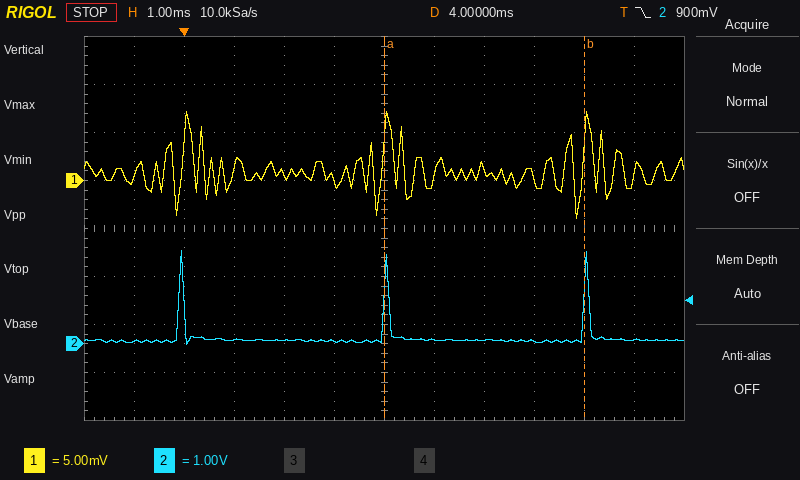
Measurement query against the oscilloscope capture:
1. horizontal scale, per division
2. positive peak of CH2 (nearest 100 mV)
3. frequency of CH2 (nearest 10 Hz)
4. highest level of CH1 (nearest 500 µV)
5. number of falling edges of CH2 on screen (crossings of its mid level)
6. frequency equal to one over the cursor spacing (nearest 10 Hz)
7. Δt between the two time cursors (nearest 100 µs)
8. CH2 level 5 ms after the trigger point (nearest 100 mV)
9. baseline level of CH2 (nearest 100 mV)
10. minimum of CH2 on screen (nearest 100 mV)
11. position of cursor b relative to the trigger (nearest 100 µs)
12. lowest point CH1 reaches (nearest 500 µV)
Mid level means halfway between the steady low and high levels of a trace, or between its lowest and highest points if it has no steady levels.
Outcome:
1 ms
1.9 V
250 Hz
7.0 mV
3
250 Hz
4.0 ms
100 mV
100 mV
0.0 V
+8.0 ms
-4.0 mV
